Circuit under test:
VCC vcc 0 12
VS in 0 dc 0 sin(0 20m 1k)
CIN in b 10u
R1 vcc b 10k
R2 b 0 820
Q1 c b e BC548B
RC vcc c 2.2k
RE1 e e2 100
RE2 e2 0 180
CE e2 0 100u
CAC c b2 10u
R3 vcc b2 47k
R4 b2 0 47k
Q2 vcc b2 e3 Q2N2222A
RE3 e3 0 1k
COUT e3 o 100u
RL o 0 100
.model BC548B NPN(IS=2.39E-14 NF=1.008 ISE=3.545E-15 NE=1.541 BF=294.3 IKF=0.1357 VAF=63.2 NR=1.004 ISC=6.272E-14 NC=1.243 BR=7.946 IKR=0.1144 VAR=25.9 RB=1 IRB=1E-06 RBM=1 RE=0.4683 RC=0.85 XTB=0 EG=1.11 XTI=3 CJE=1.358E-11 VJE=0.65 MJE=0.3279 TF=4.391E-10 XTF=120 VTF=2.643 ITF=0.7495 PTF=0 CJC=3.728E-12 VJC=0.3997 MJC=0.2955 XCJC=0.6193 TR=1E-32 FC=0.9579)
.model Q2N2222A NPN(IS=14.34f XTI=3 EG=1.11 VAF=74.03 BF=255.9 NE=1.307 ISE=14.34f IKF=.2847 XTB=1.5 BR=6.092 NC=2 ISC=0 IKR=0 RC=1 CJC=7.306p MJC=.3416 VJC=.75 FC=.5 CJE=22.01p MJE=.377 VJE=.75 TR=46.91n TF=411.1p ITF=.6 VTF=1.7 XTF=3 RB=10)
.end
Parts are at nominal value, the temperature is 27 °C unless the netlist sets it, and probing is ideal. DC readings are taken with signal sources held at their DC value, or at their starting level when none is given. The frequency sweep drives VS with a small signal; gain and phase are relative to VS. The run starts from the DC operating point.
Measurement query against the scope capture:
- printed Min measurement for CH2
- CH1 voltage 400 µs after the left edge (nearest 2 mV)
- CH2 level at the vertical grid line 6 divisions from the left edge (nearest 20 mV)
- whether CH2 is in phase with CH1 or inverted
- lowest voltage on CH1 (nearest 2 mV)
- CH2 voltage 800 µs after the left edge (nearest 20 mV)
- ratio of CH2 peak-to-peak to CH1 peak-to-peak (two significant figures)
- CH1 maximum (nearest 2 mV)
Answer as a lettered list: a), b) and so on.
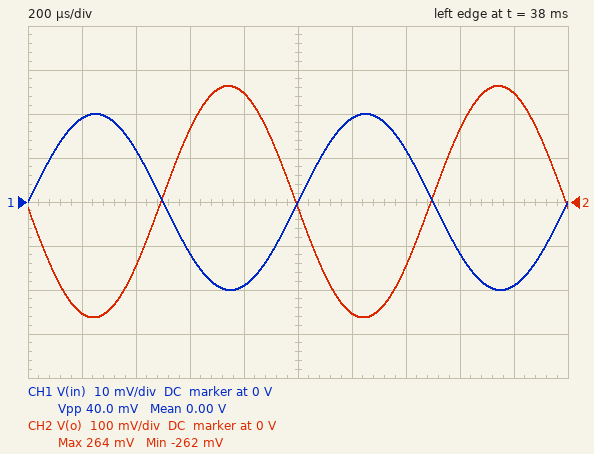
a) -262 mV
b) 12 mV
c) -260 mV
d) inverted
e) -20 mV
f) 240 mV
g) 13
h) 20 mV
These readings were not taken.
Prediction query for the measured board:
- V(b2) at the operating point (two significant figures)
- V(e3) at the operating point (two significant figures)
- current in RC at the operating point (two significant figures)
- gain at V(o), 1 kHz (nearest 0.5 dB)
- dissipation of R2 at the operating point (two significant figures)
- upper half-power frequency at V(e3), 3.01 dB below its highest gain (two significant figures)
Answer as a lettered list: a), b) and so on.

a) 5.4 V
b) 4.7 V
c) 970 µA
d) 22.5 dB
e) 1.0 mW
f) 7.7 MHz
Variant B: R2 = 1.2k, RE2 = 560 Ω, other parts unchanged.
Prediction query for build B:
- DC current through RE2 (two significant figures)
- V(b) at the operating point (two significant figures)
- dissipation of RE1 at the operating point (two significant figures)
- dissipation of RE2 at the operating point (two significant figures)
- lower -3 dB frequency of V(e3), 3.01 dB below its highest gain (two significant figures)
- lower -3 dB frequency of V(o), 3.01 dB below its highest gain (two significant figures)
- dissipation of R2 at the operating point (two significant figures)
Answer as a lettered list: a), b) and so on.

a) 980 µA
b) 1.3 V
c) 96 µW
d) 540 µW
e) 22 Hz
f) 29 Hz
g) 1.4 mW
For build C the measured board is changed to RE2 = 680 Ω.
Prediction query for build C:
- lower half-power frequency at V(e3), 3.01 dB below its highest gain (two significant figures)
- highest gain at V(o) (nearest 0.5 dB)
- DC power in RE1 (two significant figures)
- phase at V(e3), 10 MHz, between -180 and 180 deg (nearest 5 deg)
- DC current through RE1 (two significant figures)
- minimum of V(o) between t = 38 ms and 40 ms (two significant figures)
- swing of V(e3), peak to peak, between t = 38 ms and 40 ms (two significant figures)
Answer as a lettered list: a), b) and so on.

a) 25 Hz
b) 20.0 dB
c) 15 µW
d) 120 deg
e) 380 µA
f) -200 mV
g) 400 mV
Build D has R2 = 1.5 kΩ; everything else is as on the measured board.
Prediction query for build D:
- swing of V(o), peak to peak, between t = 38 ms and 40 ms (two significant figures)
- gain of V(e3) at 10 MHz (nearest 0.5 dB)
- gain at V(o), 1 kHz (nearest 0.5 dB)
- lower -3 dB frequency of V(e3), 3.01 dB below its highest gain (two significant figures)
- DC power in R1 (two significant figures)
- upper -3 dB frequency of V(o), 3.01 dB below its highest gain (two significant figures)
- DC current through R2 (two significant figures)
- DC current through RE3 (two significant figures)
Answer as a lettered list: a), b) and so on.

a) 610 mV
b) 19.5 dB
c) 24.0 dB
d) 25 Hz
e) 11 mW
f) 7.4 MHz
g) 1.0 mA
h) 4.7 mA
